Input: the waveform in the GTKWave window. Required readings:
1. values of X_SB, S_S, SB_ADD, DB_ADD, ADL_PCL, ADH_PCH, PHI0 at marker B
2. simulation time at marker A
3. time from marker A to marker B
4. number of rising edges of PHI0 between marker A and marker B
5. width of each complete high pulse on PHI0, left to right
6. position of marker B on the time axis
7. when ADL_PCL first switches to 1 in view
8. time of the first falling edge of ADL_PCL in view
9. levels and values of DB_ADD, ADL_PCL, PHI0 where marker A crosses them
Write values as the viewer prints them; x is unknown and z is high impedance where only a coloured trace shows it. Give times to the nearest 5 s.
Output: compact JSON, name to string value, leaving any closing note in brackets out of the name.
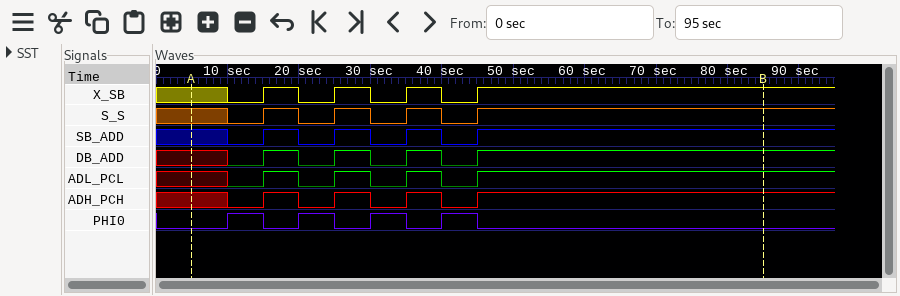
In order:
{"values of X_SB, S_S, SB_ADD, DB_ADD, ADL_PCL, ADH_PCH, PHI0 at marker B": "X_SB=1, S_S=1, SB_ADD=1, DB_ADD=1, ADL_PCL=1, ADH_PCH=1, PHI0=0", "simulation time at marker A": "5 s", "time from marker A to marker B": "80 s", "number of rising edges of PHI0 between marker A and marker B": "4", "width of each complete high pulse on PHI0, left to right": "5 s, 5 s, 5 s, 5 s", "position of marker B on the time axis": "85 s", "when ADL_PCL first switches to 1 in view": "15 s", "time of the first falling edge of ADL_PCL in view": "20 s", "levels and values of DB_ADD, ADL_PCL, PHI0 where marker A crosses them": "DB_ADD=x, ADL_PCL=x, PHI0=0"}
